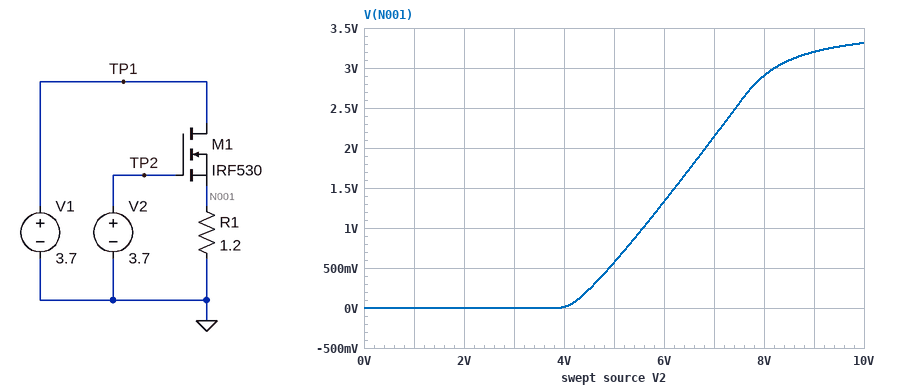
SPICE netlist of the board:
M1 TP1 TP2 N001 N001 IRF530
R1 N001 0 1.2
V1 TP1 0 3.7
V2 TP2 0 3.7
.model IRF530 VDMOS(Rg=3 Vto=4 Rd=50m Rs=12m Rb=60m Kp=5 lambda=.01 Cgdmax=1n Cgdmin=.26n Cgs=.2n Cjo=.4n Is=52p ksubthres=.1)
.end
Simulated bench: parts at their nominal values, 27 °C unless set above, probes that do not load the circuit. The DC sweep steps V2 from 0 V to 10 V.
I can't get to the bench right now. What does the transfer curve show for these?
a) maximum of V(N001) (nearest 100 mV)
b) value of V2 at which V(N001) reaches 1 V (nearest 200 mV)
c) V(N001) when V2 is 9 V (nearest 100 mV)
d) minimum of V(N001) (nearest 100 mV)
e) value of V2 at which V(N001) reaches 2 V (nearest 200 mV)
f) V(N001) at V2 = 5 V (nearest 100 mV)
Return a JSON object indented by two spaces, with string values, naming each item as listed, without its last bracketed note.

{
  "maximum of V(N001)": "3.3 V",
  "value of V2 at which V(N001) reaches 1 V": "5.6 V",
  "V(N001) when V2 is 9 V": "3.2 V",
  "minimum of V(N001)": "0 V",
  "value of V2 at which V(N001) reaches 2 V": "6.8 V",
  "V(N001) at V2 = 5 V": "600 mV"
}
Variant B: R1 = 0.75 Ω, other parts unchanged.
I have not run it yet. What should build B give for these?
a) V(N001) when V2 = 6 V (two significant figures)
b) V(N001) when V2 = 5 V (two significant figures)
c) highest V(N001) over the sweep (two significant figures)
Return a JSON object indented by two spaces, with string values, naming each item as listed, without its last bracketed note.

{
  "V(N001) when V2 = 6 V": "1.2 V",
  "V(N001) when V2 = 5 V": "490 mV",
  "highest V(N001) over the sweep": "3.1 V"
}
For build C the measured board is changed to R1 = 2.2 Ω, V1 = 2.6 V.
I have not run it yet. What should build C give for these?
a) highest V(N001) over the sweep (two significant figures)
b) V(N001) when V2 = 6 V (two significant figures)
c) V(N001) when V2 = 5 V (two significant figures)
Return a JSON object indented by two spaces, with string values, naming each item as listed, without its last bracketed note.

{
  "highest V(N001) over the sweep": "2.5 V",
  "V(N001) when V2 = 6 V": "1.5 V",
  "V(N001) when V2 = 5 V": "660 mV"
}
